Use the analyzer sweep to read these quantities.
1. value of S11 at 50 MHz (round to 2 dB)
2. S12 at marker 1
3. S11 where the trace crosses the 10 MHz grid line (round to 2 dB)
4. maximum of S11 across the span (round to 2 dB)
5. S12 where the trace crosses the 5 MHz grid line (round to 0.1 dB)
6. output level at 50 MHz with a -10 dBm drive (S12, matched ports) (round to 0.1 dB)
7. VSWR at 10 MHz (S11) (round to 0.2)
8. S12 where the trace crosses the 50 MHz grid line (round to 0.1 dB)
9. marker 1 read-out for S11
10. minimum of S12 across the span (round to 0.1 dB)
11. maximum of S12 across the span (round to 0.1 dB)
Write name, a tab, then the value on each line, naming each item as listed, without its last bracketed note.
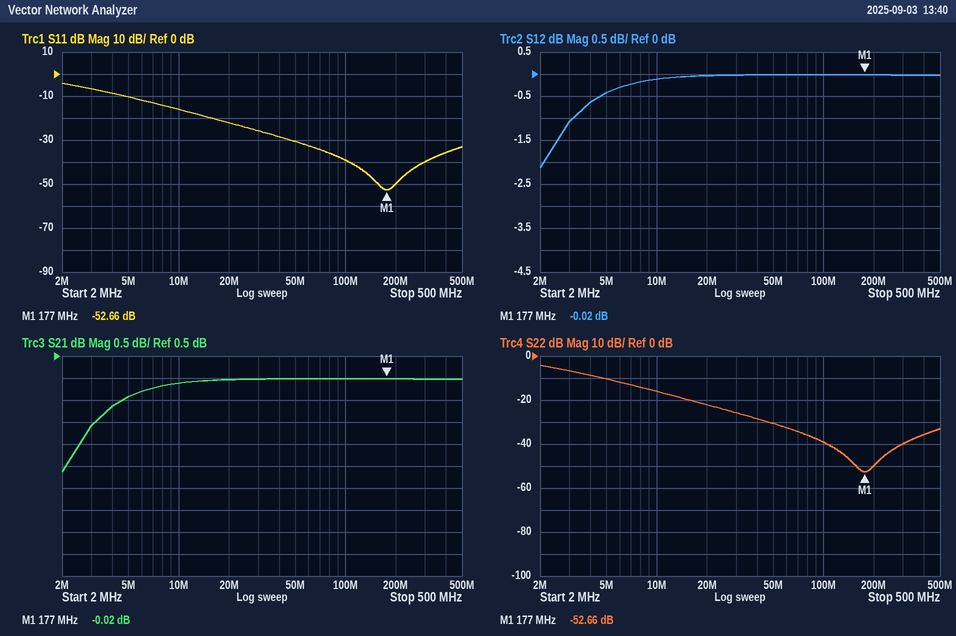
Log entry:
value of S11 at 50 MHz	-30 dB
S12 at marker 1	-0.02 dB
S11 where the trace crosses the 10 MHz grid line	-16 dB
maximum of S11 across the span	-4 dB
S12 where the trace crosses the 5 MHz grid line	-0.4 dB
output level at 50 MHz with a -10 dBm drive (S12, matched ports)	-10.0 dBm
VSWR at 10 MHz (S11)	1.4
S12 where the trace crosses the 50 MHz grid line	0.0 dB
marker 1 read-out for S11	-52.66 dB
minimum of S12 across the span	-2.1 dB
maximum of S12 across the span	0.0 dB
